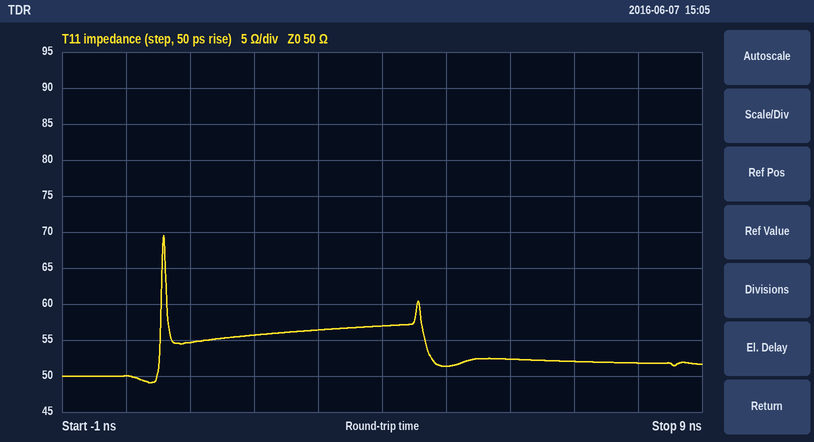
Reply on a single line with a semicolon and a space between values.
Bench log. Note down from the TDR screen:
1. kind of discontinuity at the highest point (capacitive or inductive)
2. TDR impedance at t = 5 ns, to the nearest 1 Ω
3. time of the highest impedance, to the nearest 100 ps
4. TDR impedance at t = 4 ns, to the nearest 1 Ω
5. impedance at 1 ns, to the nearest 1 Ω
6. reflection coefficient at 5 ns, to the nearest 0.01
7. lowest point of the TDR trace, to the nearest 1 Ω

inductive; 51 Ω; 600 ps; 57 Ω; 55 Ω; +0.01; 49 Ω
